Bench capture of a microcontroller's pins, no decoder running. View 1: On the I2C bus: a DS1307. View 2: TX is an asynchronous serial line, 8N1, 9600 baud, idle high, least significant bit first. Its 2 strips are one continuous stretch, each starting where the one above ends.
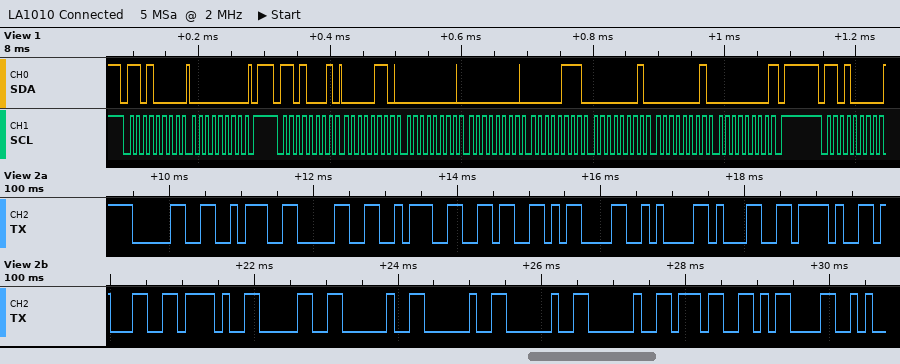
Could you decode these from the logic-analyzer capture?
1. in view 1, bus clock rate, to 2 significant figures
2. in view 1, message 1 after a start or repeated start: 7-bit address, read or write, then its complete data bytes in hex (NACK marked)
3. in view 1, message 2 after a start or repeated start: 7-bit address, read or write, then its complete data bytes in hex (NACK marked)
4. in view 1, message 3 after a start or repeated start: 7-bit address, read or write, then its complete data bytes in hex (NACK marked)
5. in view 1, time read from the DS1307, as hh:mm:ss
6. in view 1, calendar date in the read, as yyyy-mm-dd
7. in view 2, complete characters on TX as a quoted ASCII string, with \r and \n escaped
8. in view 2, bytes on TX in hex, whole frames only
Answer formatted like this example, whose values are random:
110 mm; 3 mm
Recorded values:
100 kHz; 0x68 write: 00; 0x68 read: 06 00 00 07 01 01 00 NACK; 0x68 write; 00:00:06; 2000-01-01; "0:0:6\r\n1/1/0    7\r"; 30 3A 30 3A 36 0D 0A 31 2F 31 2F 30 20 20 20 20 37 0D
